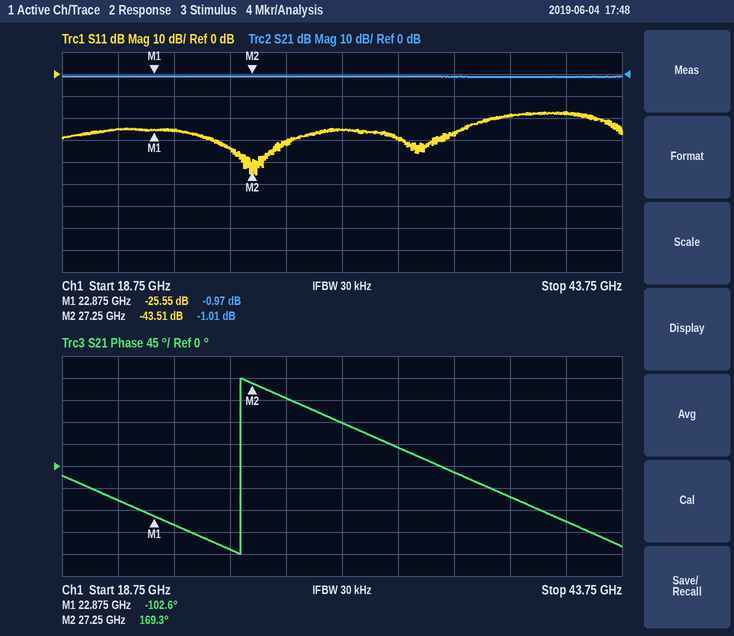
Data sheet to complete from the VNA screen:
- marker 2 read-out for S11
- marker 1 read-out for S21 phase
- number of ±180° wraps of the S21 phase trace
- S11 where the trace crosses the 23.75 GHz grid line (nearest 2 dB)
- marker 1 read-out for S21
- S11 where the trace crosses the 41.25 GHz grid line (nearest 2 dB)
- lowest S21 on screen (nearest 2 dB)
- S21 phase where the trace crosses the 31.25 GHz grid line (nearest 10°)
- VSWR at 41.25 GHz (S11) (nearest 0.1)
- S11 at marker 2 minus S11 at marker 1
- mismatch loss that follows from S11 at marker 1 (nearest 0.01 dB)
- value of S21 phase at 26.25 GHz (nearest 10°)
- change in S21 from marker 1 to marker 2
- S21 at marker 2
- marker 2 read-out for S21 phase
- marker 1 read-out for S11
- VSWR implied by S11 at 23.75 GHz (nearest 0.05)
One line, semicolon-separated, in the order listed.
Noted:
-43.51 dB; -102.6°; 1; -26 dB; -0.97 dB; -18 dB; -2 dB; 90°; 1.3; -17.96 dB; 0.01 dB; -170°; -0.04 dB; -1.01 dB; 169.3°; -25.55 dB; 1.10
